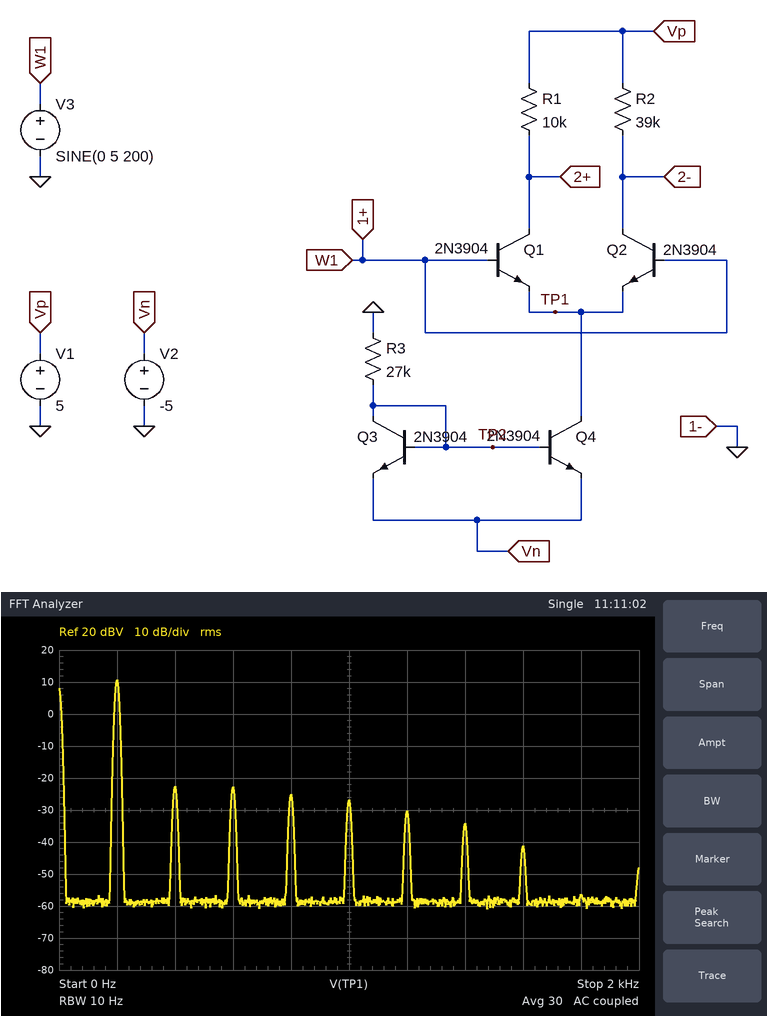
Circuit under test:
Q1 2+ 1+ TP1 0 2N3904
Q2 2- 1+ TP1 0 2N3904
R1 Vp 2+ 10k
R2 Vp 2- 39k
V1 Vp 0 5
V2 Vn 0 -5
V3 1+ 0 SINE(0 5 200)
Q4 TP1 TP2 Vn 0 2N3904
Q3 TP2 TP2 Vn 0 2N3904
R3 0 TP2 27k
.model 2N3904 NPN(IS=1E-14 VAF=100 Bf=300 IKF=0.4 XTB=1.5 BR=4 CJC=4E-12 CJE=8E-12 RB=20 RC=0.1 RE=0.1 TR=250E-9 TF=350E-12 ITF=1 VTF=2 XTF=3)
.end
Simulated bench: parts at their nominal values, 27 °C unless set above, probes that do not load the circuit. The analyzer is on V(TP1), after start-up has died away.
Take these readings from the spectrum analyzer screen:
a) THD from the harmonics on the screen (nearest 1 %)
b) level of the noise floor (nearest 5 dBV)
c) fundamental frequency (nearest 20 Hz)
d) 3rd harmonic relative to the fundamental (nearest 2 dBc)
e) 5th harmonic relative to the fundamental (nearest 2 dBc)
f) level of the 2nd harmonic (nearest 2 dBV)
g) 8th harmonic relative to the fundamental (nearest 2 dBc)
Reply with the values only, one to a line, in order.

4 %
-60 dBV
200 Hz
-34 dBc
-38 dBc
-22 dBV
-52 dBc
